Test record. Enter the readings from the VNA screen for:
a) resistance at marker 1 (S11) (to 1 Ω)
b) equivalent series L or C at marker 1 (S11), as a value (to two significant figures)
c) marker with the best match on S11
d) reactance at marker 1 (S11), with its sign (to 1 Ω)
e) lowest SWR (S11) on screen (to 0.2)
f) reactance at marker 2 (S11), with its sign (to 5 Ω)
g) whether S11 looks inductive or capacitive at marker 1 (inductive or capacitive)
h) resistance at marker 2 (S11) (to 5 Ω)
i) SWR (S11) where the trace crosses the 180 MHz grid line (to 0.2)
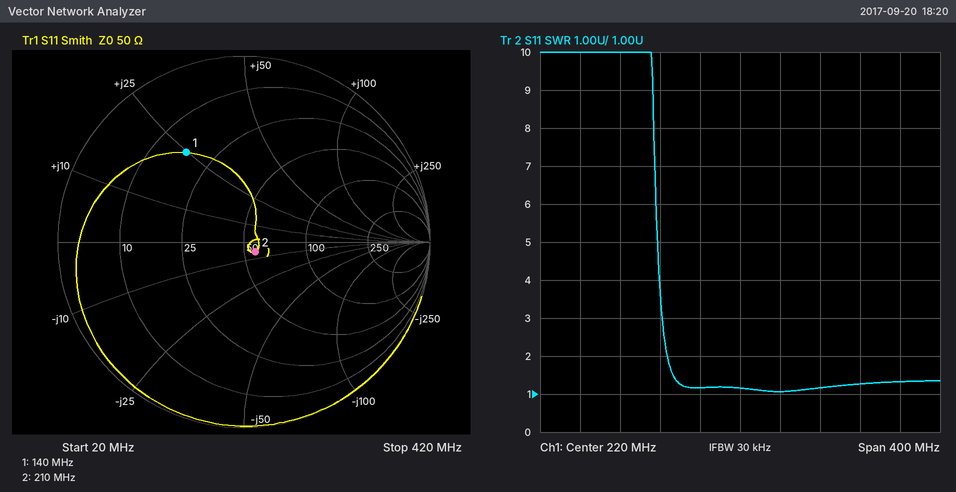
17 Ω
28 nH
marker 2
+25 Ω
1.0
-5 Ω
inductive
55 Ω
1.2
